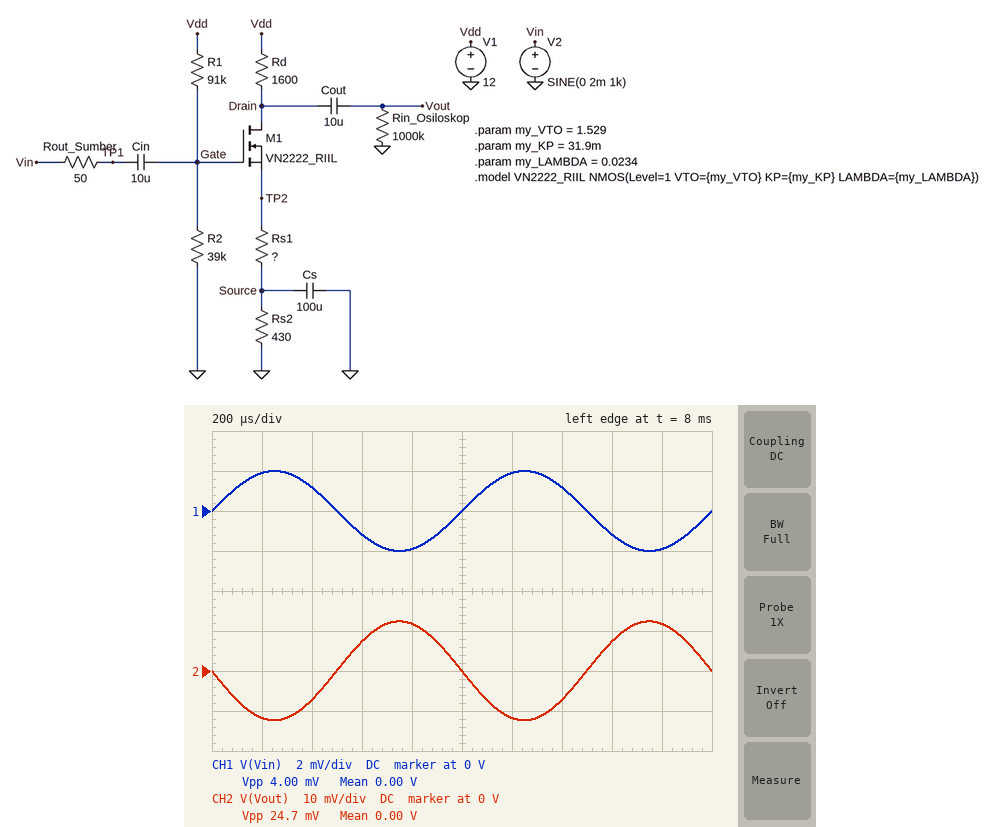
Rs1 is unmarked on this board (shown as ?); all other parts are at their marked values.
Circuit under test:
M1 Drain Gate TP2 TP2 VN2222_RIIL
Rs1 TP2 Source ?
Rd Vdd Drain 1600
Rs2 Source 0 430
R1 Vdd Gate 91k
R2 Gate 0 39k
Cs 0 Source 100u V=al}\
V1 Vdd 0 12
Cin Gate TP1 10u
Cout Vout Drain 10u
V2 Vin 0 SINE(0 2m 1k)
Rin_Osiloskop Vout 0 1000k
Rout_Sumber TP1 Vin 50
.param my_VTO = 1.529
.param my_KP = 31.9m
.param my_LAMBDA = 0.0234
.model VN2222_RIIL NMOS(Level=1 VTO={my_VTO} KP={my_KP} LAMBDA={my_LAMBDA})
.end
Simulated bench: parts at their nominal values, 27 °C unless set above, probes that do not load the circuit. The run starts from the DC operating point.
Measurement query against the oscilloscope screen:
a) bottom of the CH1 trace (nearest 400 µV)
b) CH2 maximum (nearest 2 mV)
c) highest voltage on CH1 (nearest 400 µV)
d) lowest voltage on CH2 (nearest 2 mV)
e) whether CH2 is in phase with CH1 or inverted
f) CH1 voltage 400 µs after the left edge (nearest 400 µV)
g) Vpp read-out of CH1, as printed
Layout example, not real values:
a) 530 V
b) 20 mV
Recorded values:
a) -2.0 mV
b) 12 mV
c) 2.0 mV
d) -12 mV
e) inverted
f) 1.2 mV
g) 4.00 mV
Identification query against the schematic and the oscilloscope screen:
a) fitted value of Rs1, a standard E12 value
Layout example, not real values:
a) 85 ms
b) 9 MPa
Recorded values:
a) 180 Ω
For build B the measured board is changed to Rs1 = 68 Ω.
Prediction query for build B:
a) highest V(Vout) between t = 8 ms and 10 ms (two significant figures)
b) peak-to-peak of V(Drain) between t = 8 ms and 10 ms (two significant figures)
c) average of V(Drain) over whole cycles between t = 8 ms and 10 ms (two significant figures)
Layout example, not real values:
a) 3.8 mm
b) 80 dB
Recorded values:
a) 23 mV
b) 45 mV
c) 6.7 V
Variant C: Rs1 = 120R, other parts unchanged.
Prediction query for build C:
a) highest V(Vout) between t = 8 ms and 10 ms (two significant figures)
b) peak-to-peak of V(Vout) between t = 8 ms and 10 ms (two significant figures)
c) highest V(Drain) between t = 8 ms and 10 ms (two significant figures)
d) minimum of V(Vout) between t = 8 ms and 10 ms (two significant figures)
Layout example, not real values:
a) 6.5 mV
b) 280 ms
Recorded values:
a) 16 mV
b) 33 mV
c) 7.2 V
d) -16 mV
